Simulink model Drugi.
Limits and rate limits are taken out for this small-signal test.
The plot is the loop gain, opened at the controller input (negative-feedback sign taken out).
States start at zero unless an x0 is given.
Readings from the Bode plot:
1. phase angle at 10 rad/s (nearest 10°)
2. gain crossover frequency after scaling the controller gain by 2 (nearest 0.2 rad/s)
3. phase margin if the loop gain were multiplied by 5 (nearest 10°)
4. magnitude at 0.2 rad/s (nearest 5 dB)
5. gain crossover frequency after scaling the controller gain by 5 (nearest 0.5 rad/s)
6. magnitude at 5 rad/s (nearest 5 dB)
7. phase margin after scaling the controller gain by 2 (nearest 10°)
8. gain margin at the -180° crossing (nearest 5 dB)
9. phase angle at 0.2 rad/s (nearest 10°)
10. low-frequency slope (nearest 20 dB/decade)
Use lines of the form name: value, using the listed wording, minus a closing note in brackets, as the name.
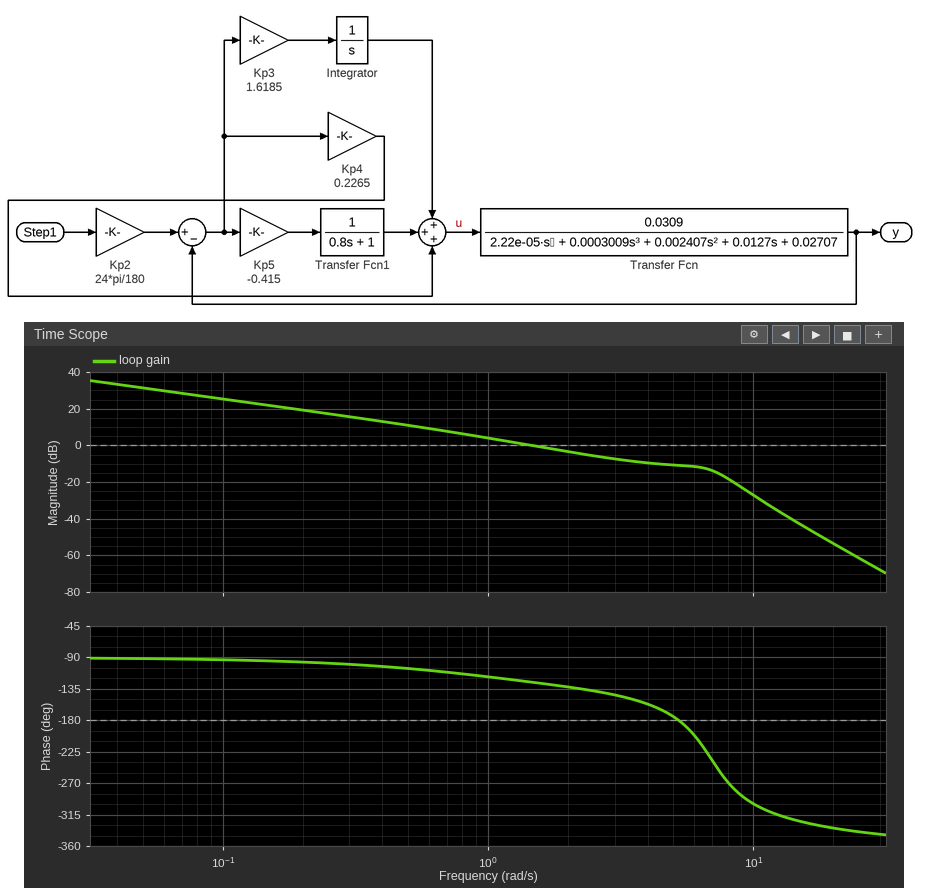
phase angle at 10 rad/s: -300°
gain crossover frequency after scaling the controller gain by 2: 2.6 rad/s
phase margin if the loop gain were multiplied by 5: -60°
magnitude at 0.2 rad/s: 20 dB
gain crossover frequency after scaling the controller gain by 5: 7.0 rad/s
magnitude at 5 rad/s: -10 dB
phase margin after scaling the controller gain by 2: 40°
gain margin at the -180° crossing: 10 dB
phase angle at 0.2 rad/s: -100°
low-frequency slope: -20 dB/decade
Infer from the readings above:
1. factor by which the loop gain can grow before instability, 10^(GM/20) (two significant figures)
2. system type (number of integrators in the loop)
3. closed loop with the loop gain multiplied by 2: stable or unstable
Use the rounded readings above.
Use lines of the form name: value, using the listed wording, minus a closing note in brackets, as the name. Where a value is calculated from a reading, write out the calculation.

factor by which the loop gain can grow before instability, 10^(GM/20): 10^(10 / 20) = 3.2
system type: 1
closed loop with the loop gain multiplied by 2: stable or unstable: stable
